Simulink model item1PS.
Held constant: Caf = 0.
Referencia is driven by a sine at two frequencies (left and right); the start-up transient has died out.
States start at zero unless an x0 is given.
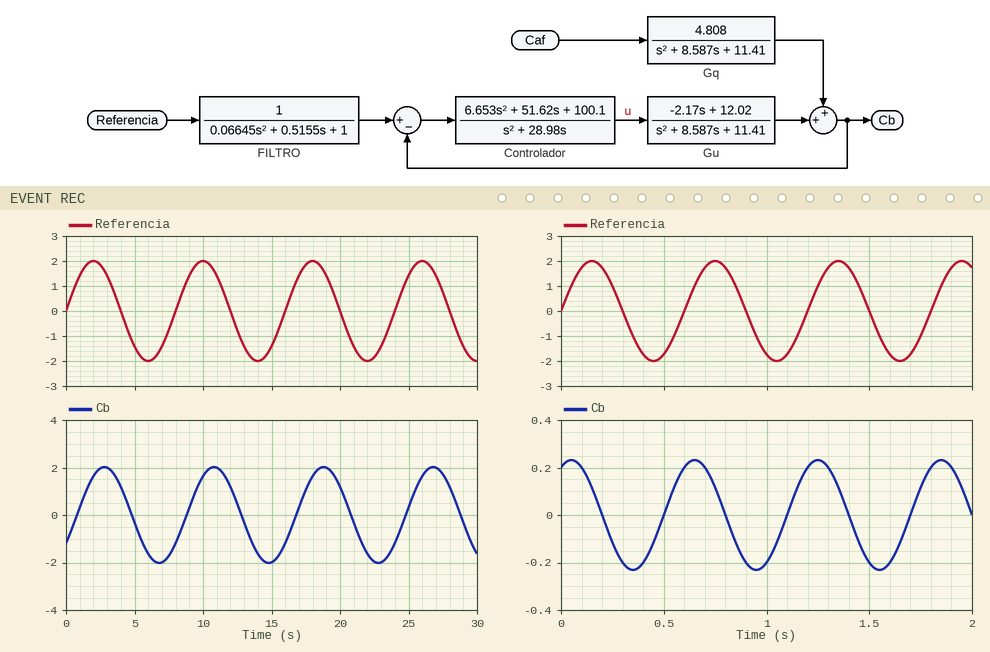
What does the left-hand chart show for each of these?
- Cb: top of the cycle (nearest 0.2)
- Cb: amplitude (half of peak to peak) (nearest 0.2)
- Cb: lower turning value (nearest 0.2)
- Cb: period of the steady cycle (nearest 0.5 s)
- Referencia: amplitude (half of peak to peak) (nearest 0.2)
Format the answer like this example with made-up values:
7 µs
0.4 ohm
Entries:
2.0
2.0
-2.0
8.0 s
2.0
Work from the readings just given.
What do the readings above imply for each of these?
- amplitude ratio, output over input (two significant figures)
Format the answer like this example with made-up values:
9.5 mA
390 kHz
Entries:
1.0
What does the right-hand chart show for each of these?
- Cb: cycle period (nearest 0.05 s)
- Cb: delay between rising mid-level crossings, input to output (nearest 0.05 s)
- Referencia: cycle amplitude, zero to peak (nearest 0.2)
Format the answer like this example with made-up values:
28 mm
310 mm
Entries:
0.60 s
0.50 s
2.0
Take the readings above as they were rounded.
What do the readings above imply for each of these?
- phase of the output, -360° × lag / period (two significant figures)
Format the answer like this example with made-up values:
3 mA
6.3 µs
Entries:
-300°
